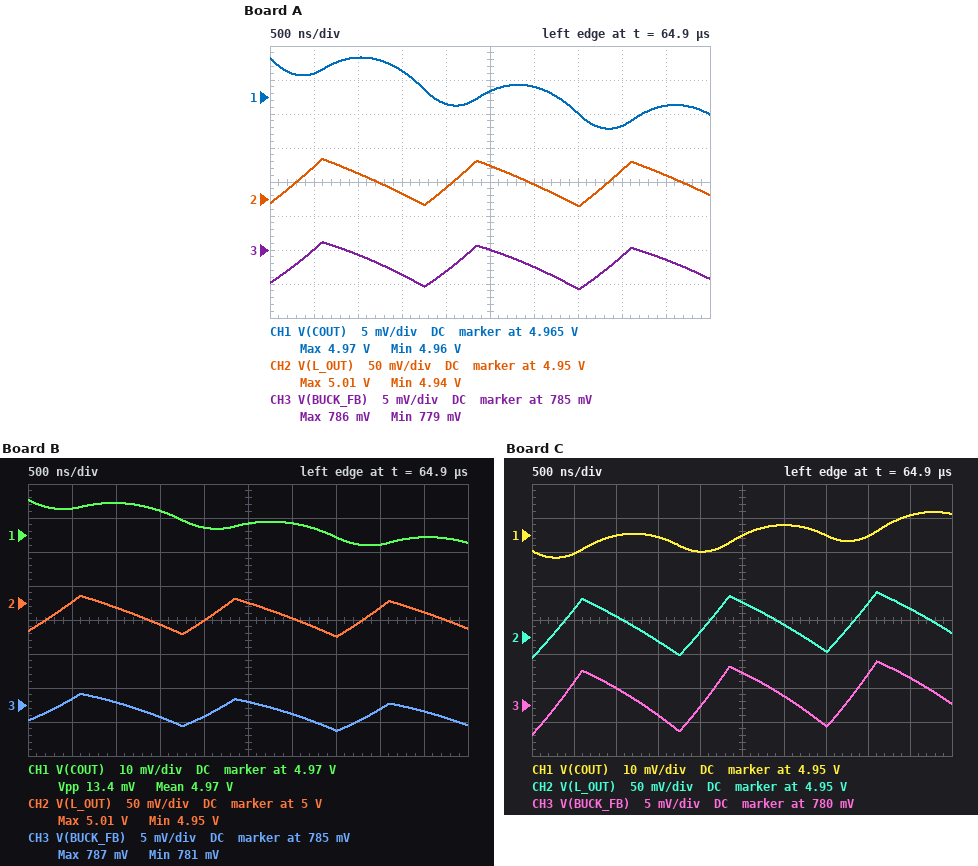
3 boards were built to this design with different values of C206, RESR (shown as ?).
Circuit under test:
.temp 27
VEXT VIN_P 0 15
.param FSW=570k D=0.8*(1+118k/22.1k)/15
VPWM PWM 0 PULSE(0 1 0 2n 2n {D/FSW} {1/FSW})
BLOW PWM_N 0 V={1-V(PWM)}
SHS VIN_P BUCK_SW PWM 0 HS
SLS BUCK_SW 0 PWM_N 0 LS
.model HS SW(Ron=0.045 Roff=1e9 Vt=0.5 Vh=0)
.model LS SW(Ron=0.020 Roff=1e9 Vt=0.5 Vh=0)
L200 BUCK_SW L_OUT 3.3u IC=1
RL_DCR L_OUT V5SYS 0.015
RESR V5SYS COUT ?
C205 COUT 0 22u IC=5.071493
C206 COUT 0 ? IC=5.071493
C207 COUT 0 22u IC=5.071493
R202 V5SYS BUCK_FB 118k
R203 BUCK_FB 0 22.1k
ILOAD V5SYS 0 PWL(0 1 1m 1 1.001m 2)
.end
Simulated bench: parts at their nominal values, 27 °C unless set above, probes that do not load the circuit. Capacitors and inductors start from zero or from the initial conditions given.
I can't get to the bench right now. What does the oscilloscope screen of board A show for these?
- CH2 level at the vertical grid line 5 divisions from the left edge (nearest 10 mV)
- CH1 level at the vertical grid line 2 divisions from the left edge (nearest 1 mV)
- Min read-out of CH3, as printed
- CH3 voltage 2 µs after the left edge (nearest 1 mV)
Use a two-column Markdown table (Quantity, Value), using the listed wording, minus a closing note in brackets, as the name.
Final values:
| Quantity | Value |
|---|---|
| CH2 level at the vertical grid line 5 divisions from the left edge | 5.00 V |
| CH1 level at the vertical grid line 2 divisions from the left edge | 4.971 V |
| Min read-out of CH3, as printed | 779 mV |
| CH3 voltage 2 µs after the left edge | 782 mV |
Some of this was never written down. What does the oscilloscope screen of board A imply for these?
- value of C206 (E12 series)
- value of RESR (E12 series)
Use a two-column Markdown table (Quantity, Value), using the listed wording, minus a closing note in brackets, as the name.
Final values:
| Quantity | Value |
|---|---|
| value of C206 | 39 µF |
| value of RESR | 0.022 Ω |
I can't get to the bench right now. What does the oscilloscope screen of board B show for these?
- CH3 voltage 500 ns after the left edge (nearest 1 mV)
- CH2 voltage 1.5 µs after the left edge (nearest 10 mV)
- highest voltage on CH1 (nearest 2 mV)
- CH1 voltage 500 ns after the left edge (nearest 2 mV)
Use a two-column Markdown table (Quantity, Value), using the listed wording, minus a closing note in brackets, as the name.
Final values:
| Quantity | Value |
|---|---|
| CH3 voltage 500 ns after the left edge | 786 mV |
| CH2 voltage 1.5 µs after the left edge | 4.97 V |
| highest voltage on CH1 | 4.980 V |
| CH1 voltage 500 ns after the left edge | 4.978 V |
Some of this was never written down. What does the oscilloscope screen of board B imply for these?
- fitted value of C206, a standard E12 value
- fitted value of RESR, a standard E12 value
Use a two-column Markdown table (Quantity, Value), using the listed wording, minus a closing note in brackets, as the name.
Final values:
| Quantity | Value |
|---|---|
| fitted value of C206, a standard E12 value | 47 µF |
| fitted value of RESR, a standard E12 value | 0.015 Ω |
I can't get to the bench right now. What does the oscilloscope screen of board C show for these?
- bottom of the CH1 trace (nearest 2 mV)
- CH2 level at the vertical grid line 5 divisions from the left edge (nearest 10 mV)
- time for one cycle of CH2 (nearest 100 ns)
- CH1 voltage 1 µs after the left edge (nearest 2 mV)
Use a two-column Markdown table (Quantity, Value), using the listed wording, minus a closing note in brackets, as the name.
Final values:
| Quantity | Value |
|---|---|
| bottom of the CH1 trace | 4.944 V |
| CH2 level at the vertical grid line 5 divisions from the left edge | 5.00 V |
| time for one cycle of CH2 | 1.7 µs |
| CH1 voltage 1 µs after the left edge | 4.950 V |
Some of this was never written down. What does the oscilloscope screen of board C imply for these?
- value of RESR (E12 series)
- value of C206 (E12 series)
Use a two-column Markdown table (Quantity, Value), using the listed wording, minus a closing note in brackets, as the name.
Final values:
| Quantity | Value |
|---|---|
| value of RESR | 0.033 Ω |
| value of C206 | 18 µF |
